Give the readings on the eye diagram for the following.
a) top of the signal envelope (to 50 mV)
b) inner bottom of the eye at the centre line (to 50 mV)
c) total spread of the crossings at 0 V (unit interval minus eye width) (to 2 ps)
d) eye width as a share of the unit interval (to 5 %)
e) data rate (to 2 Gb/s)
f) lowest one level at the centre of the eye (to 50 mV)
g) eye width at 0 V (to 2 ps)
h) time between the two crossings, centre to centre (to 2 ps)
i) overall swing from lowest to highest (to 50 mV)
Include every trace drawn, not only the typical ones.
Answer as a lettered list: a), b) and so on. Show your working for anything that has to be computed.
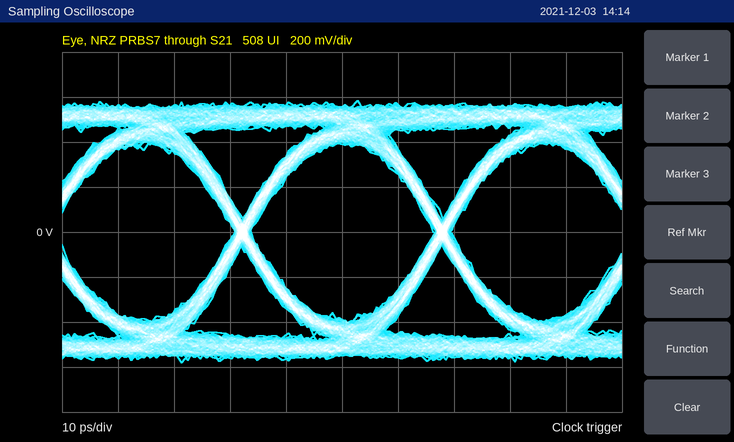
a) 600 mV
b) -400 mV
c) 4 ps
d) 32 ps / 36 ps ≈ 88.9 %, so 90 % to the nearest 5 %
e) 28 Gb/s
f) 400 mV
g) 32 ps
h) 36 ps
i) 1.15 V
